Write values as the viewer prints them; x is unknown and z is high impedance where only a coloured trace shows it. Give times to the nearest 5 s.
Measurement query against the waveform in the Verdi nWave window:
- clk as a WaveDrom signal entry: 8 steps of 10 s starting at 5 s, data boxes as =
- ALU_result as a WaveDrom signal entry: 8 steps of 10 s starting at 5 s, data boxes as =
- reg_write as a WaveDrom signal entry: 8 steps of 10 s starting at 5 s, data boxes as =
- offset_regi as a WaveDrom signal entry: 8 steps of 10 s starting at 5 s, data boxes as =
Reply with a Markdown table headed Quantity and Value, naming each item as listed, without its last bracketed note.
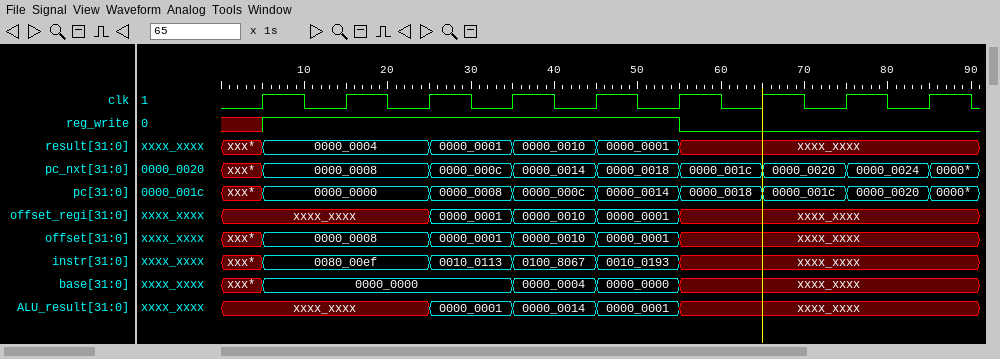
| Quantity | Value |
|---|---|
| clk as a WaveDrom signal entry: 8 steps of 10 s starting at 5 s, data boxes as = | {name: 'clk', wave: 'p.......'} |
| ALU_result as a WaveDrom signal entry: 8 steps of 10 s starting at 5 s, data boxes as = | {name: 'ALU_result', wave: 'x.===x..', data: '0000_0001 0000_0014 0000_0001'} |
| reg_write as a WaveDrom signal entry: 8 steps of 10 s starting at 5 s, data boxes as = | {name: 'reg_write', wave: '1....0..'} |
| offset_regi as a WaveDrom signal entry: 8 steps of 10 s starting at 5 s, data boxes as = | {name: 'offset_regi', wave: 'x.===x..', data: '0000_0001 0000_0010 0000_0001'} |
